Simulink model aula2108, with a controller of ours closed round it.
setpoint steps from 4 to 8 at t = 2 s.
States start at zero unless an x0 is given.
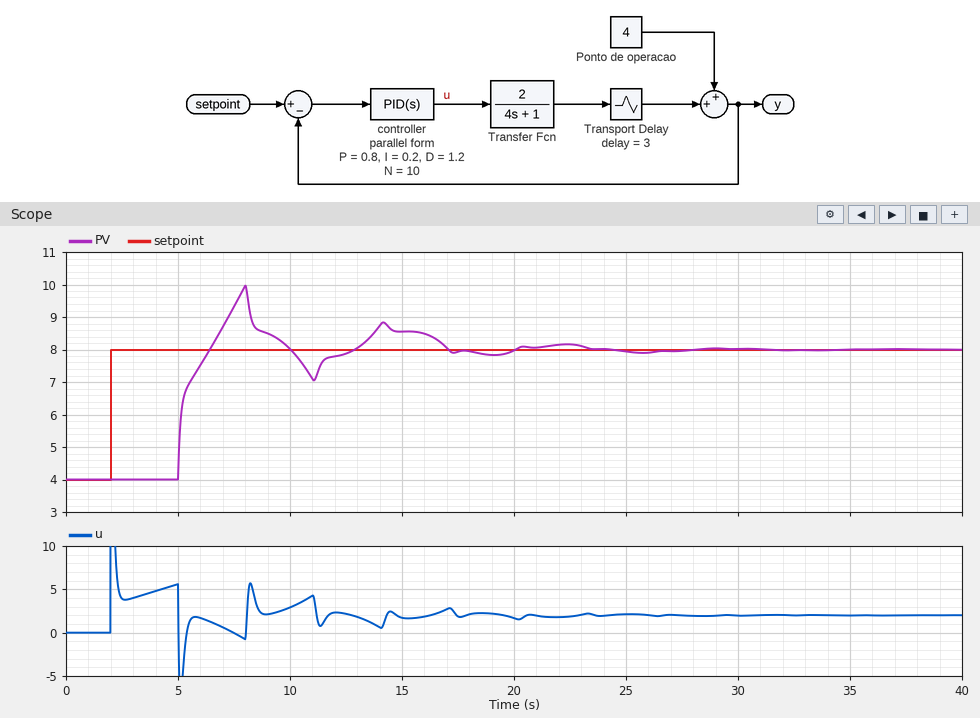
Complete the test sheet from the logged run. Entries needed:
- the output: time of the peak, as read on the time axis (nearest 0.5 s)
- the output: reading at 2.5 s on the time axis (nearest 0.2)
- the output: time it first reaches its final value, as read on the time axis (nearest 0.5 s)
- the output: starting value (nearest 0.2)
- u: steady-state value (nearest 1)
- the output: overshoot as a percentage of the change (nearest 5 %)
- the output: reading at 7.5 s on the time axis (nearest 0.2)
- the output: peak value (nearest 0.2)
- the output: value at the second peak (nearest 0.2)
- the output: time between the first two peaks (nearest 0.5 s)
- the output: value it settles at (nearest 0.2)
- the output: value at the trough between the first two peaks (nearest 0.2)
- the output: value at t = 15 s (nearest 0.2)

8.0 s
4.0
6.5 s
4.0
2
50 %
9.4
10.0
8.8
6.0 s
8.0
7.0
8.6
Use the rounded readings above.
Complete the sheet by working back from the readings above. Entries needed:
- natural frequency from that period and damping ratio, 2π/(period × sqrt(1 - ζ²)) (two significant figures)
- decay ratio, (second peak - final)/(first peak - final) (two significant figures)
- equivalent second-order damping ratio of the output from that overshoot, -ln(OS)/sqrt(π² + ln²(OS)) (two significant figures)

1.1 rad/s
0.40
0.22
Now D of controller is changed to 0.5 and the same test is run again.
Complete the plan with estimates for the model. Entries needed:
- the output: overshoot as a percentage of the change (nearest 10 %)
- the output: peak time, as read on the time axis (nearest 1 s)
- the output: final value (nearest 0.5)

40 %
10 s
8.0
